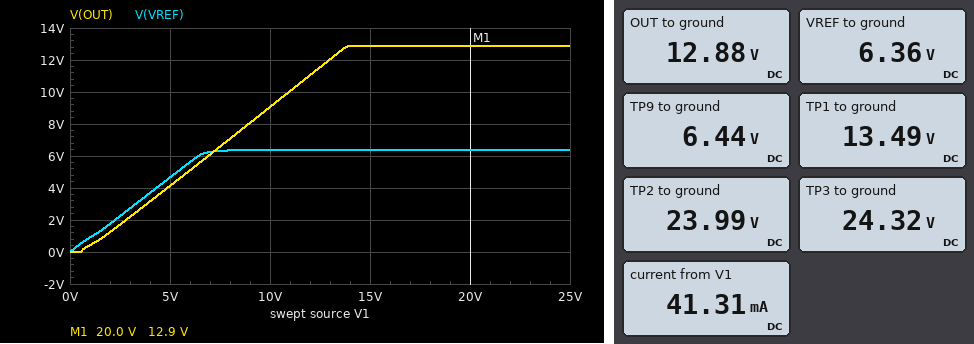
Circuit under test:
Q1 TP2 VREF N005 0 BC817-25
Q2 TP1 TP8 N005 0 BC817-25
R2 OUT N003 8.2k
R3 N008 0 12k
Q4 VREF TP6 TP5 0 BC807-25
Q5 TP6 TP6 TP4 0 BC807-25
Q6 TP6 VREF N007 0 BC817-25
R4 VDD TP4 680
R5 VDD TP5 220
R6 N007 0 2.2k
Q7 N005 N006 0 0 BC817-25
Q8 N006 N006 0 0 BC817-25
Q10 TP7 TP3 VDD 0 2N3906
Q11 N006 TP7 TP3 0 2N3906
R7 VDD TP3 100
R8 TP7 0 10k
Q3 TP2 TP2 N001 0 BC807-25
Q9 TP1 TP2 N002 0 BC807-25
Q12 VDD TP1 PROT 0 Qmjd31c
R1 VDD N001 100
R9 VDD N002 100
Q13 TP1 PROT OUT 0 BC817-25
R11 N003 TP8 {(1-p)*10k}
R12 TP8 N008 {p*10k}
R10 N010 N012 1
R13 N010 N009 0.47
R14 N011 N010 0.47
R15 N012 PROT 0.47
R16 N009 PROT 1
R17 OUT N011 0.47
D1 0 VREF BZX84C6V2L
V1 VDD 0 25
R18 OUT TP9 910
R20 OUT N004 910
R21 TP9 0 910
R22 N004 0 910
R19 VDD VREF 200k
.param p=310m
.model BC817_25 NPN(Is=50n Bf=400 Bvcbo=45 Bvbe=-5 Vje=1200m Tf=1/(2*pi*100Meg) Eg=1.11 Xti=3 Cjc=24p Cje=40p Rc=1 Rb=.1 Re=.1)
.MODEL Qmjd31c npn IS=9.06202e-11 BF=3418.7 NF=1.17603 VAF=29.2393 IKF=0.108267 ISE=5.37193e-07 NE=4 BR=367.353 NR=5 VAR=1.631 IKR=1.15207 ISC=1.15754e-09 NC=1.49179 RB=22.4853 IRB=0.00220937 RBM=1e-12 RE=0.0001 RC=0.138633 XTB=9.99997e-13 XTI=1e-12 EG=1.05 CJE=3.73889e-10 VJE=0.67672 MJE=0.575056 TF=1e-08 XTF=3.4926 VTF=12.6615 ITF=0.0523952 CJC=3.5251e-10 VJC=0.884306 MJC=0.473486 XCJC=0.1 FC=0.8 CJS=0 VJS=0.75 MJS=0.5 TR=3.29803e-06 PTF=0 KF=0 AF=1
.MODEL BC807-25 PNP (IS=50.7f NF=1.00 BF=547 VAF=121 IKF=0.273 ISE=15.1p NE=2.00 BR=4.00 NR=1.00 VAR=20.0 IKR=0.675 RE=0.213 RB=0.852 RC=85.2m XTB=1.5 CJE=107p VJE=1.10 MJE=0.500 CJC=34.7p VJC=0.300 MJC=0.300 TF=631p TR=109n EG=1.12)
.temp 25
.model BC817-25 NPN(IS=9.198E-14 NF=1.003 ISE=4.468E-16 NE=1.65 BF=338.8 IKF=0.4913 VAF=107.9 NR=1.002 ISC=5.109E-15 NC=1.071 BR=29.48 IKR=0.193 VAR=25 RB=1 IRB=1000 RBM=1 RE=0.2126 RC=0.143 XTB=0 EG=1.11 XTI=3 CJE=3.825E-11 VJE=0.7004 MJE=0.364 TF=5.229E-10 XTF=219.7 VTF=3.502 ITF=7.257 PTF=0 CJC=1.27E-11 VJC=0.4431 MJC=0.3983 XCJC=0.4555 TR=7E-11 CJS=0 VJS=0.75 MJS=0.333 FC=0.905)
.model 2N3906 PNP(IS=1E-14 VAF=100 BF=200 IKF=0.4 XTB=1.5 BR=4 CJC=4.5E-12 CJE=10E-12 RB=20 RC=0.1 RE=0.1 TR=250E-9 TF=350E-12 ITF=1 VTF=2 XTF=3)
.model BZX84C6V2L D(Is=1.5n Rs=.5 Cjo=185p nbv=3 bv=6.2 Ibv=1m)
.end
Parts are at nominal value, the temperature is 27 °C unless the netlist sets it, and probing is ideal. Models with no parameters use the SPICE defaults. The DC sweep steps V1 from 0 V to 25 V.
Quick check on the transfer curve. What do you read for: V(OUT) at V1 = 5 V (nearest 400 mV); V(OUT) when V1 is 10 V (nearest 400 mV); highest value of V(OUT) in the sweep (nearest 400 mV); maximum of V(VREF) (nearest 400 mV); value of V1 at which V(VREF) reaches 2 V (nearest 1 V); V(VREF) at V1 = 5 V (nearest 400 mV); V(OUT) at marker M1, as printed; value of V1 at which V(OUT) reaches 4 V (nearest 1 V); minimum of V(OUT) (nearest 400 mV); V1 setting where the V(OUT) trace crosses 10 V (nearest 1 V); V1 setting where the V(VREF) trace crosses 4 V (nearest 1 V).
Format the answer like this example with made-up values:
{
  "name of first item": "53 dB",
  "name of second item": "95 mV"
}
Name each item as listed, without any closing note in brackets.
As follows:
{
  "V(OUT) at V1 = 5 V": "4.0 V",
  "V(OUT) when V1 is 10 V": "9.2 V",
  "highest value of V(OUT) in the sweep": "12.8 V",
  "maximum of V(VREF)": "6.4 V",
  "value of V1 at which V(VREF) reaches 2 V": "2 V",
  "V(VREF) at V1 = 5 V": "4.8 V",
  "V(OUT) at marker M1, as printed": "12.9 V",
  "value of V1 at which V(OUT) reaches 4 V": "5 V",
  "minimum of V(OUT)": "0 V",
  "V1 setting where the V(OUT) trace crosses 10 V": "11 V",
  "V1 setting where the V(VREF) trace crosses 4 V": "4 V"
}
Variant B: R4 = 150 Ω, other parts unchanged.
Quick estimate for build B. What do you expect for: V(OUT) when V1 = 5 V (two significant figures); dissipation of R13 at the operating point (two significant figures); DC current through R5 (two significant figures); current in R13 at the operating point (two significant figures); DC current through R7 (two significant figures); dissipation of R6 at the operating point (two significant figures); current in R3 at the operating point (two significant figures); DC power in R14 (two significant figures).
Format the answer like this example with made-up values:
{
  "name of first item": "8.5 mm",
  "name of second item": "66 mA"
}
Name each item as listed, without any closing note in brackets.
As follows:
{
  "V(OUT) when V1 = 5 V": "4.2 V",
  "dissipation of R13 at the operating point": "24 µW",
  "DC current through R5": "1.8 mA",
  "current in R13 at the operating point": "7.2 mA",
  "DC current through R7": "6.8 mA",
  "dissipation of R6 at the operating point": "14 mW",
  "current in R3 at the operating point": "410 µA",
  "DC power in R14": "96 µW"
}
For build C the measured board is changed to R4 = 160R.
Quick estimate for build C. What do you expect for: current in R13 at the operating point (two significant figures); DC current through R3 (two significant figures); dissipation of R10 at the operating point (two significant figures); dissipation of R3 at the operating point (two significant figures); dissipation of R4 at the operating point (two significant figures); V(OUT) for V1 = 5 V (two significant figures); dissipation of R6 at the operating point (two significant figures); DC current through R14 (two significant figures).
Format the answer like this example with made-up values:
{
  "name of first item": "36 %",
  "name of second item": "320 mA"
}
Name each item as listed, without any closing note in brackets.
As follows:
{
  "current in R13 at the operating point": "7.2 mA",
  "DC current through R3": "410 µA",
  "dissipation of R10 at the operating point": "51 µW",
  "dissipation of R3 at the operating point": "2.1 mW",
  "dissipation of R4 at the operating point": "1.0 mW",
  "V(OUT) for V1 = 5 V": "4.2 V",
  "dissipation of R6 at the operating point": "14 mW",
  "DC current through R14": "14 mA"
}
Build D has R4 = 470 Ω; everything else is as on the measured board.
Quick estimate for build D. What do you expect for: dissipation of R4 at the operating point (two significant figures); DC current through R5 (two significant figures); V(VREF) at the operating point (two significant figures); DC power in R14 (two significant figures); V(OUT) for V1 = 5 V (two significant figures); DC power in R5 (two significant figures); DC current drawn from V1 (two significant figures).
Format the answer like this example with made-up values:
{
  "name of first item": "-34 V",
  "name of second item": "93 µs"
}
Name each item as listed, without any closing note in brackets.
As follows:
{
  "dissipation of R4 at the operating point": "3.1 mW",
  "DC current through R5": "5.4 mA",
  "V(VREF) at the operating point": "6.3 V",
  "DC power in R14": "99 µW",
  "V(OUT) for V1 = 5 V": "4.1 V",
  "DC power in R5": "6.5 mW",
  "DC current drawn from V1": "39 mA"
}
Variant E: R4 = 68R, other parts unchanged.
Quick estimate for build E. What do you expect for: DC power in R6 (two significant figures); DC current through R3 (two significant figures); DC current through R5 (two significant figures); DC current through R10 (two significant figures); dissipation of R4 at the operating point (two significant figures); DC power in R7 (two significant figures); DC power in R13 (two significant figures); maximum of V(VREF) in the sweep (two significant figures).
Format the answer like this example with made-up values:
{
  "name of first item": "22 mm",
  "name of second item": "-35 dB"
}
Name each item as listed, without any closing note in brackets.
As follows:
{
  "DC power in R6": "14 mW",
  "DC current through R3": "410 µA",
  "DC current through R5": "920 µA",
  "DC current through R10": "7.1 mA",
  "dissipation of R4 at the operating point": "430 µW",
  "DC power in R7": "4.6 mW",
  "DC power in R13": "24 µW",
  "maximum of V(VREF) in the sweep": "6.2 V"
}
